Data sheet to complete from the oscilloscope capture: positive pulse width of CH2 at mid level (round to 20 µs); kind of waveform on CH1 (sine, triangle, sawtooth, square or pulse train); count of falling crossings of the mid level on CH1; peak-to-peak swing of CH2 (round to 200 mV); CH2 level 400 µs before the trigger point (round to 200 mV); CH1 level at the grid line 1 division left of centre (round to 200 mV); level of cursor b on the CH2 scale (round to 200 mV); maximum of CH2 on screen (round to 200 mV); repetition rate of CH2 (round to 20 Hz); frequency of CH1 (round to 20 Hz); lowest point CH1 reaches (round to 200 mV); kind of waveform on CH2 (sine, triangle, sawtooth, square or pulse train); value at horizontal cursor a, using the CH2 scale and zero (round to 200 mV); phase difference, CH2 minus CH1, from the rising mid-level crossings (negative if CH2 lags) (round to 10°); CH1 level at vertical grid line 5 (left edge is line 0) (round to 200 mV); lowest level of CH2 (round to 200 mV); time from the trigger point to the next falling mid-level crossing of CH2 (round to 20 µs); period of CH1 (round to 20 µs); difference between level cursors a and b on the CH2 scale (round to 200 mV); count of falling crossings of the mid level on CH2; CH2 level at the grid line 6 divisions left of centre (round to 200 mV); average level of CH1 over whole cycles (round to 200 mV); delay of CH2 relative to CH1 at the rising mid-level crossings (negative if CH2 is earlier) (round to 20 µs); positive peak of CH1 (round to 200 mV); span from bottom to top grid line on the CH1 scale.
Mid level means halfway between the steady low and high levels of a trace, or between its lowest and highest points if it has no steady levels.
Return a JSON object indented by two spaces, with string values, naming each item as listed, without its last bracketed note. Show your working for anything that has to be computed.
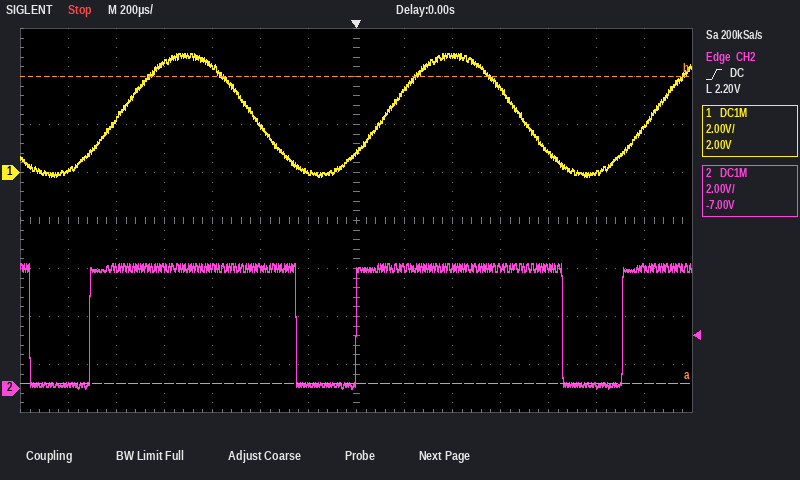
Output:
{
  "positive pulse width of CH2 at mid level": "860 µs",
  "kind of waveform on CH1": "sine",
  "count of falling crossings of the mid level on CH1": "2",
  "peak-to-peak swing of CH2": "5.2 V − (0.0 V) = 5.2 V",
  "CH2 level 400 µs before the trigger point": "5.0 V",
  "CH1 level at the grid line 1 division left of centre": "0.0 V",
  "level of cursor b on the CH2 scale": "13.0 V",
  "maximum of CH2 on screen": "5.2 V",
  "repetition rate of CH2": "900 Hz",
  "frequency of CH1": "1 / 1.12 ms ≈ 893 Hz, so 900 Hz to the nearest 20 Hz",
  "lowest point CH1 reaches": "-200 mV",
  "kind of waveform on CH2": "pulse train",
  "value at horizontal cursor a, using the CH2 scale and zero": "200 mV",
  "phase difference, CH2 minus CH1, from the rising mid-level crossings (negative if CH2 lags)": "−360° × (-120 µs) / 1.12 ms ≈ +38.6°, so +40° to the nearest 10°",
  "CH1 level at vertical grid line 5 (left edge is line 0)": "2.0 V",
  "lowest level of CH2": "0.0 V",
  "time from the trigger point to the next falling mid-level crossing of CH2": "860 µs",
  "period of CH1": "1.12 ms",
  "difference between level cursors a and b on the CH2 scale": "12.8 V",
  "count of falling crossings of the mid level on CH2": "3",
  "CH2 level at the grid line 6 divisions left of centre": "200 mV",
  "average level of CH1 over whole cycles": "(5.0 V + (-200 mV)) / 2 ≈ 2.4 V",
  "delay of CH2 relative to CH1 at the rising mid-level crossings (negative if CH2 is earlier)": "-120 µs",
  "positive peak of CH1": "5.0 V",
  "span from bottom to top grid line on the CH1 scale": "16 V"
}
